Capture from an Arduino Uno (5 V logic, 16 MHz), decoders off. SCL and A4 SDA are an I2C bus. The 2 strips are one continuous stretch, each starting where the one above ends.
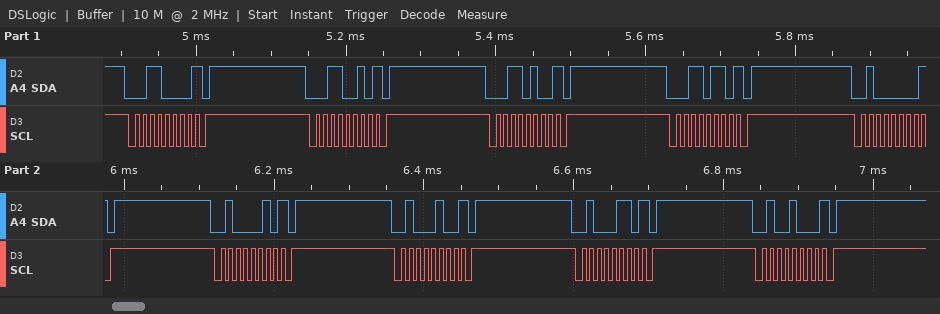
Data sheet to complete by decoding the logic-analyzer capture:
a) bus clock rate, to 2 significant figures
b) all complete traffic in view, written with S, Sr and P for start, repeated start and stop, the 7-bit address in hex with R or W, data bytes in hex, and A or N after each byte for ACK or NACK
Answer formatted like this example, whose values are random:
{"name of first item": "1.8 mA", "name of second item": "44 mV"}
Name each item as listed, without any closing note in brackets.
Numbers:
{"bus clock rate, to 2 significant figures": "100 kHz", "all complete traffic in view, written with S, Sr and P for start, repeated start and stop, the 7-bit address in hex with R or W, data bytes in hex, and A or N after each byte for ACK or NACK": "S 18W N P S 19W N P S 1AW N P S 1BW N P S 20W N P S 21W N P S 22W N P S 23W N P S 24W N P"}
